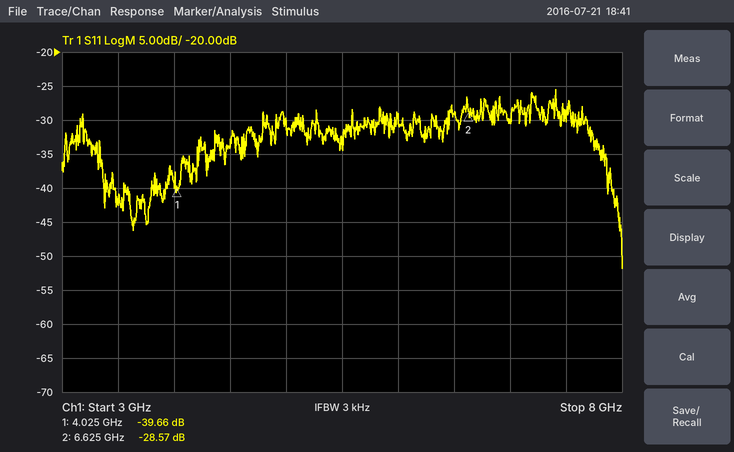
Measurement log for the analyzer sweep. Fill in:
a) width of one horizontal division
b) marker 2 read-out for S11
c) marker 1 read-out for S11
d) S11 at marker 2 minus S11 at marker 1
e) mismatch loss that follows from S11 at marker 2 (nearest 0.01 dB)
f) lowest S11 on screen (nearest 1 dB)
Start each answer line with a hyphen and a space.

- 500 MHz
- -28.57 dB
- -39.66 dB
- 11.09 dB
- 0.01 dB
- -52 dB
